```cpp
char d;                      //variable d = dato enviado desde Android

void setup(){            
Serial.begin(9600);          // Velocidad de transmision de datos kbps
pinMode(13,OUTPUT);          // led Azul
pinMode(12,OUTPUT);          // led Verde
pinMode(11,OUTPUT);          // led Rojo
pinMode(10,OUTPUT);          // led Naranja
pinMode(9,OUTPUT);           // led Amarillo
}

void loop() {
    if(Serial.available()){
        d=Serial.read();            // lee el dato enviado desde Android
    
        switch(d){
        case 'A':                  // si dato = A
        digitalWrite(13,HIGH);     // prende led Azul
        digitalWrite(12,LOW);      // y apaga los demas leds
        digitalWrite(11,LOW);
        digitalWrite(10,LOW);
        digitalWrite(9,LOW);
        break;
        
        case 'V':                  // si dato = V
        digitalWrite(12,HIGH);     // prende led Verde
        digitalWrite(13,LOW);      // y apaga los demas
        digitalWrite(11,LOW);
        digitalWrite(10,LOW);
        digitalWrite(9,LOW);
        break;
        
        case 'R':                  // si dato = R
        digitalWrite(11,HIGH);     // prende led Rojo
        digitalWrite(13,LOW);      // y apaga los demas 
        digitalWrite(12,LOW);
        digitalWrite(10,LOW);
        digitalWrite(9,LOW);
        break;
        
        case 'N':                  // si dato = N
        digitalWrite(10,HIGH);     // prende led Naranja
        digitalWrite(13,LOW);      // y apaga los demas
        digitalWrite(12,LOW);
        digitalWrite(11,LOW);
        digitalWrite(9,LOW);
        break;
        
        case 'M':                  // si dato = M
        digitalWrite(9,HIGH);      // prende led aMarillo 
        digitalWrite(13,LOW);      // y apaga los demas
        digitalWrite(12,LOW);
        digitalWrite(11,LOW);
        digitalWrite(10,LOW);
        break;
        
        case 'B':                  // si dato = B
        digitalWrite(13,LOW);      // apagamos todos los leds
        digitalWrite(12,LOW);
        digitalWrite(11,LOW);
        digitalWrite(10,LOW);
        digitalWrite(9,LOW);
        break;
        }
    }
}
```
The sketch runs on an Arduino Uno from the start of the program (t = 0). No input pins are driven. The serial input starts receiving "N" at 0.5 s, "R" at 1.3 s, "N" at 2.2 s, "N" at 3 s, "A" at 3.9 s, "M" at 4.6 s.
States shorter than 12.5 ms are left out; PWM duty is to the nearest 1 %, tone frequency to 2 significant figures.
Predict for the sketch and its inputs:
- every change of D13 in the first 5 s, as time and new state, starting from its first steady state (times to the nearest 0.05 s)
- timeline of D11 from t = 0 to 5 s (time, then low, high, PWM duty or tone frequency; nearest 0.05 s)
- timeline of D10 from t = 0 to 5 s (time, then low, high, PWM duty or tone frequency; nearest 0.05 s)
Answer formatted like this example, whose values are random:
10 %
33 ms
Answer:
0 s low; 3.9 s high; 4.6 s low
0 s low; 1.3 s high; 2.2 s low
0 s low; 0.5 s high; 1.3 s low; 2.2 s high; 3.9 s low
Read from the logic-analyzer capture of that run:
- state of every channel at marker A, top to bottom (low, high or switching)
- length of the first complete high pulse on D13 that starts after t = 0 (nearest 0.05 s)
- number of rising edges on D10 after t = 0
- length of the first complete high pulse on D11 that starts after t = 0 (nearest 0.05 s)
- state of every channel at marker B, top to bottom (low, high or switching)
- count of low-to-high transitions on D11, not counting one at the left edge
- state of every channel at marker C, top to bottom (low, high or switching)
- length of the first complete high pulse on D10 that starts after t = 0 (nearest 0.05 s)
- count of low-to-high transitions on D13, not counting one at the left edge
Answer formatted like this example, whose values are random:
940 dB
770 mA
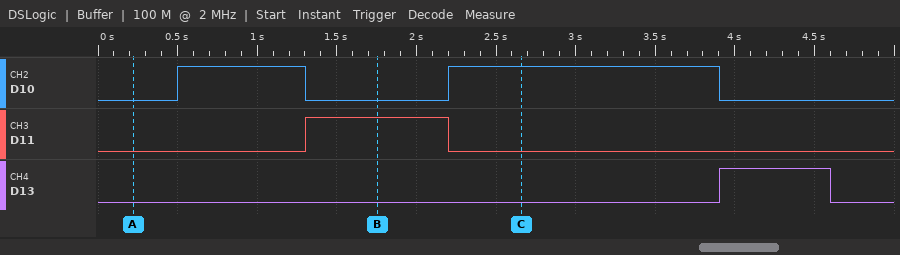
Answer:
D10 low, D11 low, D13 low
0.70 s
2
0.90 s
D10 low, D11 high, D13 low
1
D10 high, D11 low, D13 low
0.80 s
1
